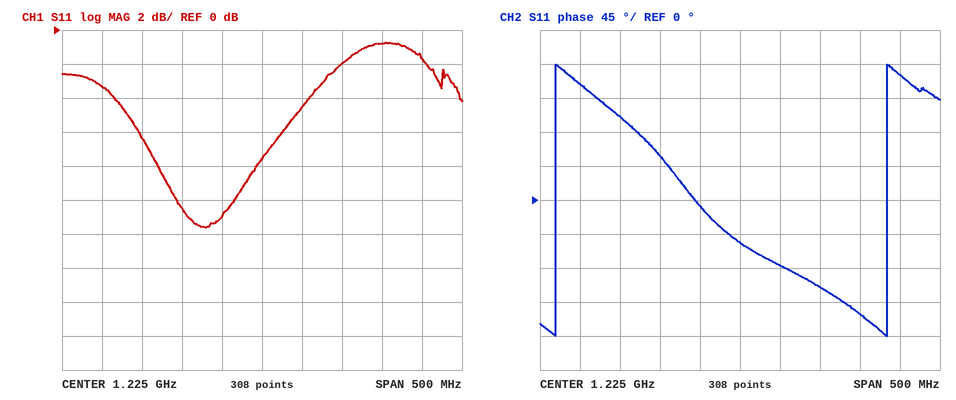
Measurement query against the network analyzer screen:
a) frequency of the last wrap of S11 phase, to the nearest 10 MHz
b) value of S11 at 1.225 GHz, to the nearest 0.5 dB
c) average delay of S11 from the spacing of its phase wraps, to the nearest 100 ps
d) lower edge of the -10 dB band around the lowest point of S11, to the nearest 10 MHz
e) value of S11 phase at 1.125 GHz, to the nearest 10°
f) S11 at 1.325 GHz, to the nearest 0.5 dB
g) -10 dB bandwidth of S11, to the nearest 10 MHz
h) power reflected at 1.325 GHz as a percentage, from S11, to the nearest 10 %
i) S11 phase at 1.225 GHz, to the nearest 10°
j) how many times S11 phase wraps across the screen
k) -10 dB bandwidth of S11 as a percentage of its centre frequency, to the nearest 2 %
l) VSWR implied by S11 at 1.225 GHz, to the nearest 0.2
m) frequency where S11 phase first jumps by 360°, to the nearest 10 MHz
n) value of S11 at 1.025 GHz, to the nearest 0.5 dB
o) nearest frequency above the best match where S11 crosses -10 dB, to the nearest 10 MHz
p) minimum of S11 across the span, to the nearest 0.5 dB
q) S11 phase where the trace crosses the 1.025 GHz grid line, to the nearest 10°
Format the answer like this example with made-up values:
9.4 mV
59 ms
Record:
1.41 GHz
-7.5 dB
2.4 ns
1.12 GHz
60°
-2.0 dB
70 MHz
60 %
-60°
2
6 %
2.4
990 MHz
-3.5 dB
1.19 GHz
-11.5 dB
150°
